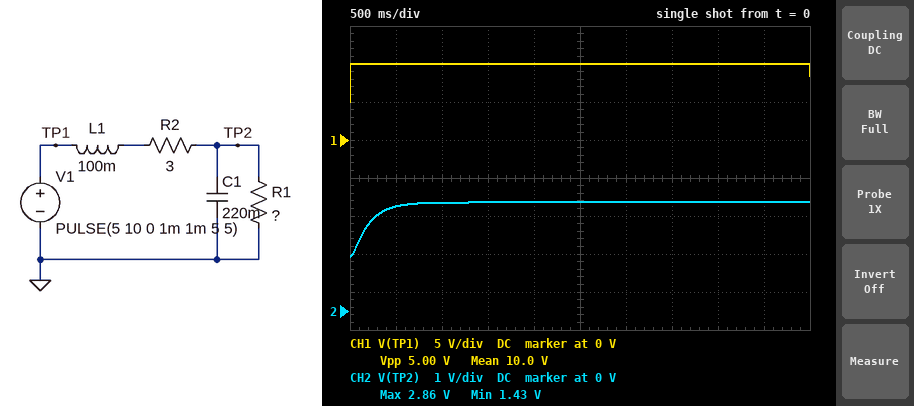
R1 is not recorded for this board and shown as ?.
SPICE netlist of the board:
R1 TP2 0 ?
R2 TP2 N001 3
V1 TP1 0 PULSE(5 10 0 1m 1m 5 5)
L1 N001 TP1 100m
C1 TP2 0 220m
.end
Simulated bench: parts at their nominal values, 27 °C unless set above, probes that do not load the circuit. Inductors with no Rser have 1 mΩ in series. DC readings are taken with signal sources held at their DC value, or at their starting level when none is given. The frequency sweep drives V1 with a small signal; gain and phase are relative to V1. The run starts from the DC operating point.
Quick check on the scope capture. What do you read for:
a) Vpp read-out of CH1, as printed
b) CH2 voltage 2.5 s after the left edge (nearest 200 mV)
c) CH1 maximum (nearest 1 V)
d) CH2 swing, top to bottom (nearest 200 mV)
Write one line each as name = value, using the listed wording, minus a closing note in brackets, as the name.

Vpp read-out of CH1, as printed = 5.00 V
CH2 voltage 2.5 s after the left edge = 2.8 V
CH1 maximum = 10 V
CH2 swing, top to bottom = 1.4 V
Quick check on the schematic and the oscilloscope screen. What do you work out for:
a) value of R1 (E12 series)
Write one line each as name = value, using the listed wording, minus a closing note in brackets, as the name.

value of R1 = 1.2 Ω
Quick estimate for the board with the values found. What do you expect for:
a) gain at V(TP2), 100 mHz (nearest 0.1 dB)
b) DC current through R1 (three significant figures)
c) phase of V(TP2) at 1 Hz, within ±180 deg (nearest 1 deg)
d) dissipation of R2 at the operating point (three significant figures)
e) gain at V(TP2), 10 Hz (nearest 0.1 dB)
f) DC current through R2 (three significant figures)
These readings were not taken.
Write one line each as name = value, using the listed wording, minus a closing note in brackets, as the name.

gain at V(TP2), 100 mHz = -10.9 dB
DC current through R1 = 1.19 A
phase of V(TP2) at 1 Hz, within ±180 deg = -61 deg
dissipation of R2 at the operating point = 4.25 W
gain at V(TP2), 10 Hz = -39.6 dB
DC current through R2 = 1.19 A
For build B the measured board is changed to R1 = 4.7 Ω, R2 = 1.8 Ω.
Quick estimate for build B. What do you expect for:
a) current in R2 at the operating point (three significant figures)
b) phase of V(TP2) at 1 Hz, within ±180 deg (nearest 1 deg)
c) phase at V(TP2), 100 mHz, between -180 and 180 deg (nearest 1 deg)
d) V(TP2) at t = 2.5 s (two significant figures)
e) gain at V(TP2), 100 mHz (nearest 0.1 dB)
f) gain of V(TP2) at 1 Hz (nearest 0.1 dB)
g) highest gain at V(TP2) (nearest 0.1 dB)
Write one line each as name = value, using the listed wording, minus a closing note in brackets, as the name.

current in R2 at the operating point = 769 mA
phase of V(TP2) at 1 Hz, within ±180 deg = -79 deg
phase at V(TP2), 100 mHz, between -180 and 180 deg = -11 deg
V(TP2) at t = 2.5 s = 7.2 V
gain at V(TP2), 100 mHz = -2.9 dB
gain of V(TP2) at 1 Hz = -8.5 dB
highest gain at V(TP2) = -2.8 dB
